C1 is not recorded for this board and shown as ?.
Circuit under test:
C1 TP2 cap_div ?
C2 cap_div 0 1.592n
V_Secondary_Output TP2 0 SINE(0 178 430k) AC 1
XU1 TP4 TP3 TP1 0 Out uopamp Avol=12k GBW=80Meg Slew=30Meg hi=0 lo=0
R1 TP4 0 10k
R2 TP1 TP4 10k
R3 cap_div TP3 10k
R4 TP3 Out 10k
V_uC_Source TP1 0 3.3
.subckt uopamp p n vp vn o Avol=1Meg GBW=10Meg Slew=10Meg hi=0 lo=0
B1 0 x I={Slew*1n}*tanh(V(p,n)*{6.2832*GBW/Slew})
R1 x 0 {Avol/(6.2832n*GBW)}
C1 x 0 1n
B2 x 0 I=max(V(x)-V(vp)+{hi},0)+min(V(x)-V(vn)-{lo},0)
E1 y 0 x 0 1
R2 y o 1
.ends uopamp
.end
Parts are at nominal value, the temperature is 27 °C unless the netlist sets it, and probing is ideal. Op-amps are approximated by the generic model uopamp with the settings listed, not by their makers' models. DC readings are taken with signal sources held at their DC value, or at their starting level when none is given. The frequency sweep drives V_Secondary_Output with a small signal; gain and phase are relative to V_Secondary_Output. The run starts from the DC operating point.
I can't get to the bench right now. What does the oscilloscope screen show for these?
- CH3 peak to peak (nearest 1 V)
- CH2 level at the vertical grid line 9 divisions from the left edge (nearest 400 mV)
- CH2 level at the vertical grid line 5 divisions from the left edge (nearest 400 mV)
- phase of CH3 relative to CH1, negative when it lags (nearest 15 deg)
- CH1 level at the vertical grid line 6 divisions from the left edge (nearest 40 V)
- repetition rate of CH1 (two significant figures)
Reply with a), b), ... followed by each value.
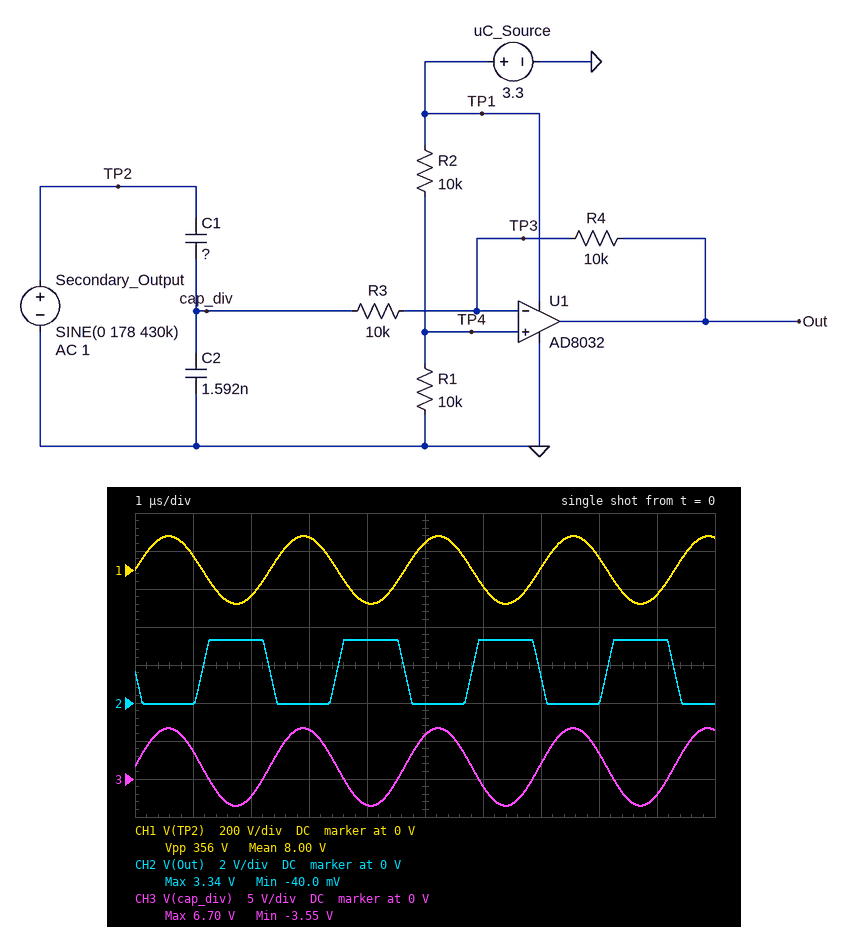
a) 10 V
b) 3.2 V
c) 0 V
d) 0 deg
e) -80 V
f) 430 kHz
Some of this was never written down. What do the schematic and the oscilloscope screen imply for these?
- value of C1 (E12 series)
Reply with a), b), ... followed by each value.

a) 47 pF
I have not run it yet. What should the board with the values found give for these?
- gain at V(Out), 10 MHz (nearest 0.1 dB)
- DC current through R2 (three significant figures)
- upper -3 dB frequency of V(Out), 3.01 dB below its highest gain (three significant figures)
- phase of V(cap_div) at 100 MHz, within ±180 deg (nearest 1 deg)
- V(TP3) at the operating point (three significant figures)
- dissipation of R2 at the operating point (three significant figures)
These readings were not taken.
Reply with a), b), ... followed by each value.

a) -31.1 dB
b) 165 µA
c) 40.0 MHz
d) 0 deg
e) 1.65 V
f) 272 µW
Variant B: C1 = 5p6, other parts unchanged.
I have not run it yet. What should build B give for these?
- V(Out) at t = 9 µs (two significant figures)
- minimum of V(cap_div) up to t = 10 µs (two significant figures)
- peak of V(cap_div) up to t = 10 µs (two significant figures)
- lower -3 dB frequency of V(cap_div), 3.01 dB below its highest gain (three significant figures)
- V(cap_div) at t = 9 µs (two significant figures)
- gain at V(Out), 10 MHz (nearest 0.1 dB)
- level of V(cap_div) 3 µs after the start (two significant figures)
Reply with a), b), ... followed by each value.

a) 2.1 V
b) 1.0 V
c) 2.3 V
d) 9.96 kHz
e) 1.2 V
f) -49.4 dB
g) 2.2 V
